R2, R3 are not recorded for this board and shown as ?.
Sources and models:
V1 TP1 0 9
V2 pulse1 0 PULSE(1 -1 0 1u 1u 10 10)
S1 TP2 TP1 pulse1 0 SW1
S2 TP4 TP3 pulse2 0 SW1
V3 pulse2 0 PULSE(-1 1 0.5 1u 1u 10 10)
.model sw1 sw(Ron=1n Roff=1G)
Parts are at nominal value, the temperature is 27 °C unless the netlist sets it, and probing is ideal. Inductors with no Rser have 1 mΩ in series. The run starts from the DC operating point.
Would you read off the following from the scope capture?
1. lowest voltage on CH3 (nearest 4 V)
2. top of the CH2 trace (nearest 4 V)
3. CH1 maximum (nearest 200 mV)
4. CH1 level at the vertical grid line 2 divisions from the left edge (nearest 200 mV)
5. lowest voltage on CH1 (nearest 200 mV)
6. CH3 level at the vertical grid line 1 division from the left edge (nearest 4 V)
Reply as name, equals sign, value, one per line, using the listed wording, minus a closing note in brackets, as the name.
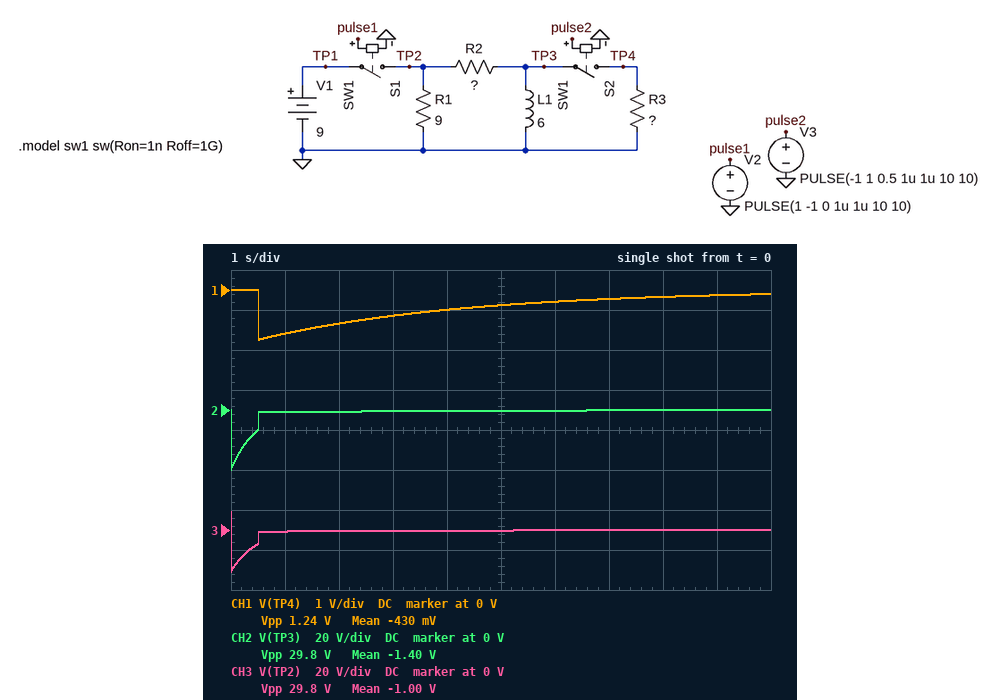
lowest voltage on CH3 = -20 V
top of the CH2 trace = 0 V
CH1 maximum = 0 V
CH1 level at the vertical grid line 2 divisions from the left edge = -800 mV
lowest voltage on CH1 = -1.2 V
CH3 level at the vertical grid line 1 division from the left edge = 0 V
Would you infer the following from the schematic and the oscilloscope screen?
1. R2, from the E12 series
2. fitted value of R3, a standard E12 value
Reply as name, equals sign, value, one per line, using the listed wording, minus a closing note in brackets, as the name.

R2, from the E12 series = 3.9 Ω
fitted value of R3, a standard E12 value = 1.8 Ω
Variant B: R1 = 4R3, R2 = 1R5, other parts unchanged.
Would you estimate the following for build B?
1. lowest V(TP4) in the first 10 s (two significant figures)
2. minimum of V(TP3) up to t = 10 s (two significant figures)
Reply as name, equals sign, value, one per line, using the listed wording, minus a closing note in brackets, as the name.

lowest V(TP4) in the first 10 s = -5.1 V
minimum of V(TP3) up to t = 10 s = -35 V
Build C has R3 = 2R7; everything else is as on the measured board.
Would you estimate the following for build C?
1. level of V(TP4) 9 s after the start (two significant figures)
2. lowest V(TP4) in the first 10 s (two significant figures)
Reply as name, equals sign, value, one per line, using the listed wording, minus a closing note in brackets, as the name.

level of V(TP4) 9 s after the start = -74 mV
lowest V(TP4) in the first 10 s = -1.8 V
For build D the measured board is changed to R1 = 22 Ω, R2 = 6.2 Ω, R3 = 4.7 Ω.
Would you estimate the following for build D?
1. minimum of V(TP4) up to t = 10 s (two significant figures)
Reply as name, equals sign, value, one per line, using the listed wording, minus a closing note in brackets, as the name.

minimum of V(TP4) up to t = 10 s = -560 mV
